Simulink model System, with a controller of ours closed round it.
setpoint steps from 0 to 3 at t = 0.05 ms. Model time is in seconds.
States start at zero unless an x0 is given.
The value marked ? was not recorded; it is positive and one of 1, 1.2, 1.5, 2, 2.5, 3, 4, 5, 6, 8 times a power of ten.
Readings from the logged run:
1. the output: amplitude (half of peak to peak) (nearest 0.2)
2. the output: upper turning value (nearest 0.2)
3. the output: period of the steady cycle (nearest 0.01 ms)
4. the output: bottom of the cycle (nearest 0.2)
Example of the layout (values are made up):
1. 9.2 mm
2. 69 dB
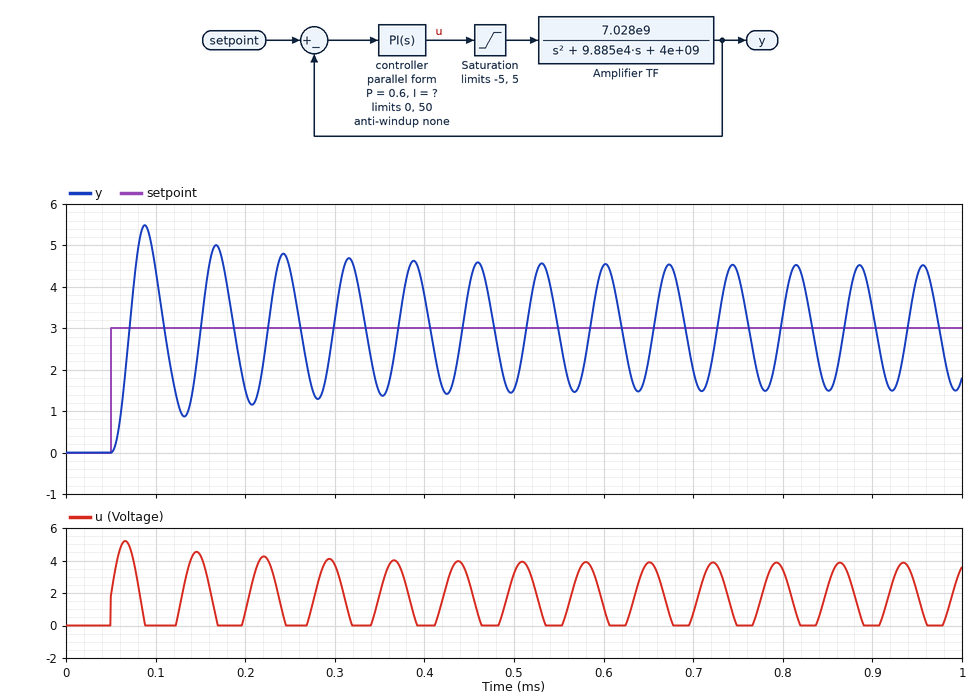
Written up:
1. 1.6
2. 4.6
3. 0.07 ms
4. 1.4
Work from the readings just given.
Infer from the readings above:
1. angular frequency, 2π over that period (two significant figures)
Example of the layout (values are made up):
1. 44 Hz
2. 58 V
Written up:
1. 90 rad/ms
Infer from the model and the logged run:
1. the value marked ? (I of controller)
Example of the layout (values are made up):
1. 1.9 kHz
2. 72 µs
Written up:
1. 120000
